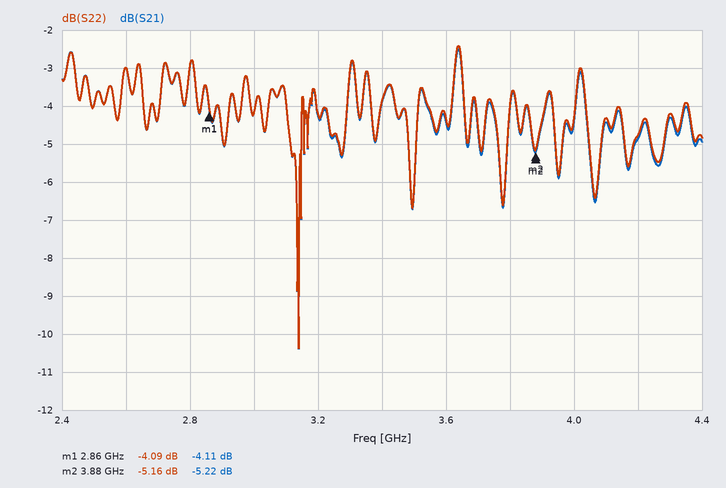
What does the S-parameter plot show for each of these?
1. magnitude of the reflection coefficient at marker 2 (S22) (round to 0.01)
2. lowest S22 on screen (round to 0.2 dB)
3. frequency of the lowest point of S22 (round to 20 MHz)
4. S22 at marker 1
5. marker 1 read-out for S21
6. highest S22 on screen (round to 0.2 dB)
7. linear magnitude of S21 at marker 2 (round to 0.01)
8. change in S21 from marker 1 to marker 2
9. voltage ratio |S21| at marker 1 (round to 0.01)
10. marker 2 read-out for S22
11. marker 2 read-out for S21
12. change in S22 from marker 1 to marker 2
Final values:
0.55
-10.4 dB
3.14 GHz
-4.09 dB
-4.11 dB
-2.4 dB
0.55
-1.11 dB
0.62
-5.16 dB
-5.22 dB
-1.07 dB
